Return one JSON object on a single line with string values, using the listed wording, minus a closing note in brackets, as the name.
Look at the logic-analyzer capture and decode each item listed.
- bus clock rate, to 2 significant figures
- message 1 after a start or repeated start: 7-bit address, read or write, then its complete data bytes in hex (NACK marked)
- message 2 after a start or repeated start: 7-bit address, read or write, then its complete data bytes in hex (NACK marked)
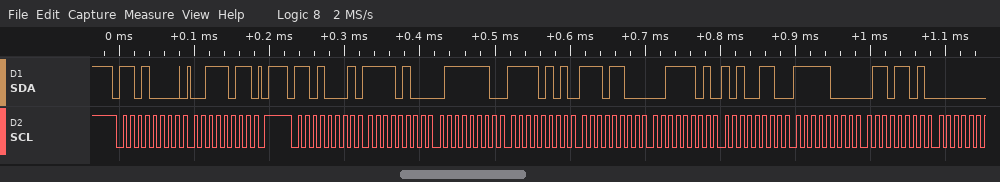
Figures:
{"bus clock rate, to 2 significant figures": "100 kHz", "message 1 after a start or repeated start: 7-bit address, read or write, then its complete data bytes in hex": "0x68 write: 3B", "message 2 after a start or repeated start: 7-bit address, read or write, then its complete data bytes in hex": "0x68 read: F4 7E F5 EC 3D A6 F8 6D"}
